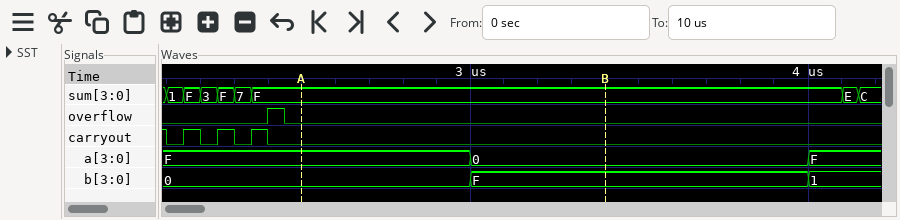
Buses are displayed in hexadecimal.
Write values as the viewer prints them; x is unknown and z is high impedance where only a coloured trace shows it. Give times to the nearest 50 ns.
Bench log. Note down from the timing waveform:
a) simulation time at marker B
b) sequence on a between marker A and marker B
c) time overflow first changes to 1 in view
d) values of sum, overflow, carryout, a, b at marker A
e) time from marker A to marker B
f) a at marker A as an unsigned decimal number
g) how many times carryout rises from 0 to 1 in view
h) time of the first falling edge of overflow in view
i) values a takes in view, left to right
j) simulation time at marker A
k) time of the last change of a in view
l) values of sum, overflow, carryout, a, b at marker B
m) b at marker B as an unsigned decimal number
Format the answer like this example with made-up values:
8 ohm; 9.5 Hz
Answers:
3400 ns; F, 0; 2400 ns; sum=F, overflow=0, carryout=0, a=F, b=0; 900 ns; 15; 3; 2450 ns; F, 0, F; 2500 ns; 4000 ns; sum=F, overflow=0, carryout=0, a=0, b=F; 15
